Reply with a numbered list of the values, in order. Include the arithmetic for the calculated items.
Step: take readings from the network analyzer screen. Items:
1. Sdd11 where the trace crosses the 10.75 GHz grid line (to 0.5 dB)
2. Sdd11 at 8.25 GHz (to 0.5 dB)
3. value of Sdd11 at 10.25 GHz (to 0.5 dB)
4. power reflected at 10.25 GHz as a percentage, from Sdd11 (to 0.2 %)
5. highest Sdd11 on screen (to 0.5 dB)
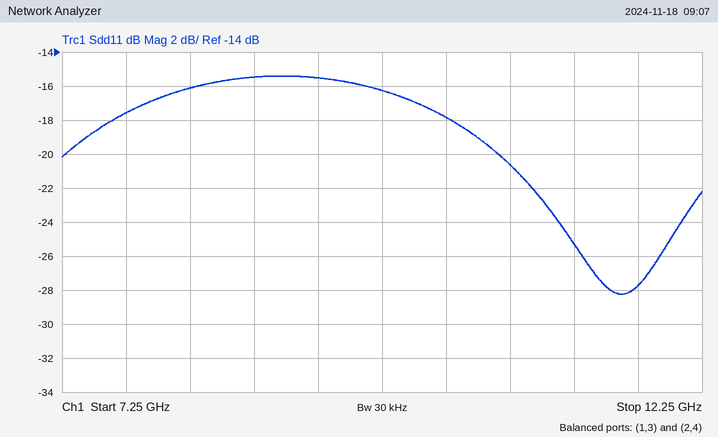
1. -20.5 dB
2. -16.0 dB
3. -18.0 dB
4. 10^(-18/10) ≈ 1.6 %
5. -15.5 dB
